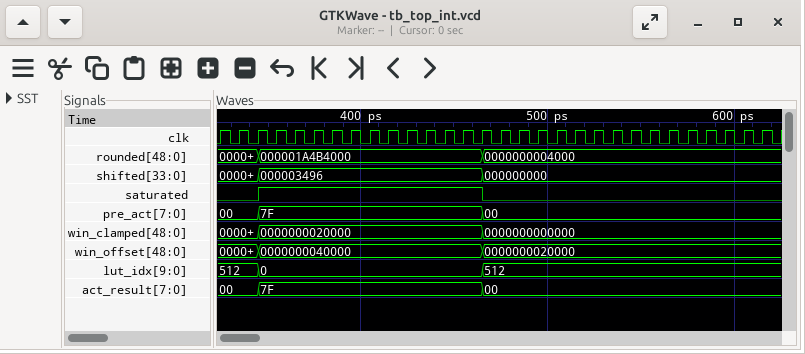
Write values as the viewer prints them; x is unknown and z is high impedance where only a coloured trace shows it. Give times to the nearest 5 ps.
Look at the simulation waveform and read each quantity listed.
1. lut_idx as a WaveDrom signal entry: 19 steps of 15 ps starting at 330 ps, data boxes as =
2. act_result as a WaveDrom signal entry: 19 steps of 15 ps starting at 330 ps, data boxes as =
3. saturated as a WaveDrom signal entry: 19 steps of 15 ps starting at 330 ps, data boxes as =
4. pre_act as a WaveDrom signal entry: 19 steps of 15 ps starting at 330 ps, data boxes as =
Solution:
{name: 'lut_idx', wave: '==.......=.........', data: '512 0 512'}
{name: 'act_result', wave: '==.......=.........', data: '00 7F 00'}
{name: 'saturated', wave: '01.......0.........'}
{name: 'pre_act', wave: '==.......=.........', data: '00 7F 00'}
